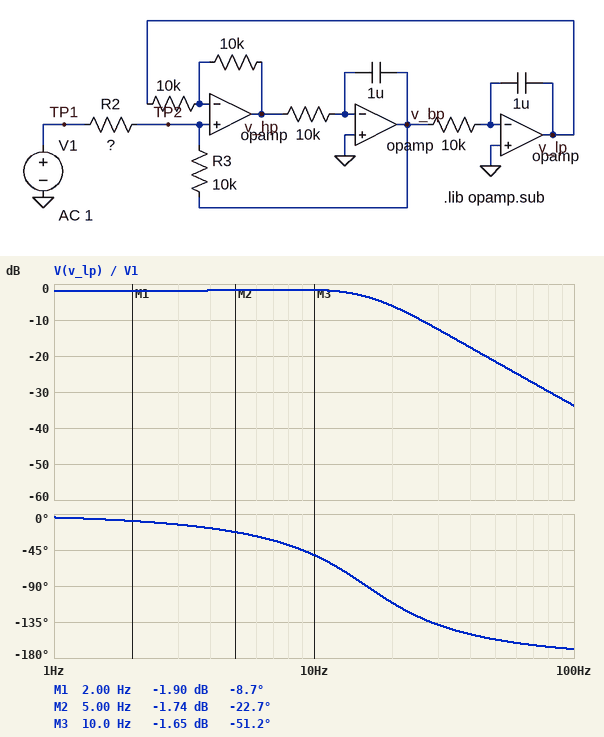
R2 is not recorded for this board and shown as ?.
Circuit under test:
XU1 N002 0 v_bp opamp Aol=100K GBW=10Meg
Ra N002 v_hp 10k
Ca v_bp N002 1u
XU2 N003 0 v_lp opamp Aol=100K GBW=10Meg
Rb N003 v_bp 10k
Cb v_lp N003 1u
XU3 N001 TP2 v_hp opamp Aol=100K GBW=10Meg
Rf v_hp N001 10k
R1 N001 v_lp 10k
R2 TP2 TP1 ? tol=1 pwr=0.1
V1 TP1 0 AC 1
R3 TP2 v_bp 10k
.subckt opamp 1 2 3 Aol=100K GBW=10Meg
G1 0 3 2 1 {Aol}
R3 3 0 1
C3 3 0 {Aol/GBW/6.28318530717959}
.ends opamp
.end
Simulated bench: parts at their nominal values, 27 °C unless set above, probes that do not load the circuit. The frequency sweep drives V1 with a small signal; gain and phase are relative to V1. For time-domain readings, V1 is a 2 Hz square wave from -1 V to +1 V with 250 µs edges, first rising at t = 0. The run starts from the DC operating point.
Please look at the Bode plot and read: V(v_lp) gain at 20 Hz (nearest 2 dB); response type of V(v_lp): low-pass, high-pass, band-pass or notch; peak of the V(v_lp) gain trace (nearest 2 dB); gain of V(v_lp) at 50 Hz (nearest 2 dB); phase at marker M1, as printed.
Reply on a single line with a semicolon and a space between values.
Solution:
-6 dB; low-pass; -2 dB; -22 dB; -8.7 deg
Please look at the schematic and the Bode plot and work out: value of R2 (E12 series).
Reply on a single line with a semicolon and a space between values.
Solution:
15 kΩ
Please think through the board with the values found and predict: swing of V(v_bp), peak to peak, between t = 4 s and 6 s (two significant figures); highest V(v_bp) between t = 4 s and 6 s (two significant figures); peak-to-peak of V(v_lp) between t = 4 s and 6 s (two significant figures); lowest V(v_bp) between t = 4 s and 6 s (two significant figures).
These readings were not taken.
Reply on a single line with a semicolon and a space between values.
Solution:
1.6 V; 800 mV; 1.9 V; -800 mV
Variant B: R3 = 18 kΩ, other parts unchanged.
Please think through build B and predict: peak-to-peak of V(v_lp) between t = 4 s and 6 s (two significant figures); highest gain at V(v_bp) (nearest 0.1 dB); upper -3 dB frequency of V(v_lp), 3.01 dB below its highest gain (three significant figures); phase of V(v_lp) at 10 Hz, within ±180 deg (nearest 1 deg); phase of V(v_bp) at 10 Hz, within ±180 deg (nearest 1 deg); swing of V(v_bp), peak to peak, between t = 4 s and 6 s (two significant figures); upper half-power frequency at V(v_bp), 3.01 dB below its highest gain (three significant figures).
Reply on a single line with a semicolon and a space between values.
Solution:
3.1 V; 1.6 dB; 18.8 Hz; -43 deg; -133 deg; 2.5 V; 24.7 Hz
